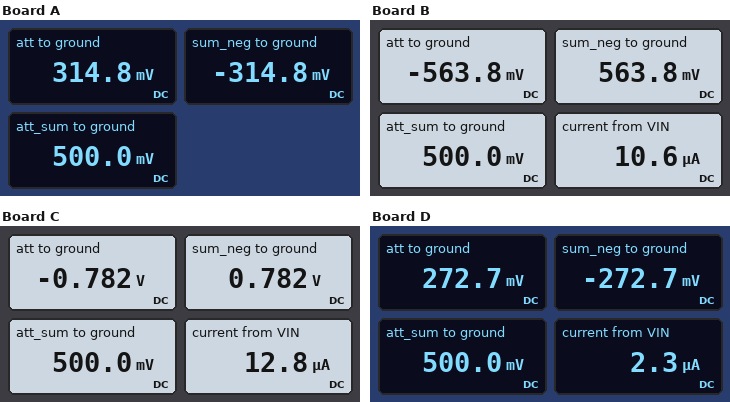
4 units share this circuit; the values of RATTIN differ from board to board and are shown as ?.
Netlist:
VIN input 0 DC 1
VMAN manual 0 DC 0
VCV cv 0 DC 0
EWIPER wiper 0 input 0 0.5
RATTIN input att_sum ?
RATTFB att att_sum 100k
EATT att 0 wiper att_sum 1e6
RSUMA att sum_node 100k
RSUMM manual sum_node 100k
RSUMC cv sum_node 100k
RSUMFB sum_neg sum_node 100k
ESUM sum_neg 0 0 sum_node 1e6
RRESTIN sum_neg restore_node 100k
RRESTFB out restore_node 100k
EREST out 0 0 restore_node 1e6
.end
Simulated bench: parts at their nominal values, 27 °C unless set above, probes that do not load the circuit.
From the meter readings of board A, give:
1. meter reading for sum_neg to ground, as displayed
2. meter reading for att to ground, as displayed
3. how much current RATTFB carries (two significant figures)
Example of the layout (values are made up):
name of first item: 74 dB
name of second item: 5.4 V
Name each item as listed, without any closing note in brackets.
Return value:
meter reading for sum_neg to ground, as displayed: -314.8 mV
meter reading for att to ground, as displayed: 314.8 mV
how much current RATTFB carries: 1.9 µA
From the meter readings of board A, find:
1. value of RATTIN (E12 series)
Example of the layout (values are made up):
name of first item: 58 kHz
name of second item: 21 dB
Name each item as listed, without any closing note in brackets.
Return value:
value of RATTIN: 270 kΩ
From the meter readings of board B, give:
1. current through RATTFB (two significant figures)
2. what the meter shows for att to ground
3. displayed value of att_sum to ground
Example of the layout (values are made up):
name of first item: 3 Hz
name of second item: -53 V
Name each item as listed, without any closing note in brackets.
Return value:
current through RATTFB: 11 µA
what the meter shows for att to ground: -563.8 mV
displayed value of att_sum to ground: 500.0 mV
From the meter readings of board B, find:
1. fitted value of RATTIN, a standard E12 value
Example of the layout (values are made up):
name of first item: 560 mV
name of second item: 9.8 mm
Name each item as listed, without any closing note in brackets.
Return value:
fitted value of RATTIN, a standard E12 value: 47 kΩ
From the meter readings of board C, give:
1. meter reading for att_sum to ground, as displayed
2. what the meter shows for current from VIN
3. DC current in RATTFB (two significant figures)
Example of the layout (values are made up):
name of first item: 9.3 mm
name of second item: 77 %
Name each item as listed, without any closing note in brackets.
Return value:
meter reading for att_sum to ground, as displayed: 500.0 mV
what the meter shows for current from VIN: 12.8 µA
DC current in RATTFB: 13 µA
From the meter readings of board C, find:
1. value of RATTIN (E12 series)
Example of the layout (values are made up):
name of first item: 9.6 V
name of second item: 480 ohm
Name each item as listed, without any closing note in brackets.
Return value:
value of RATTIN: 39 kΩ
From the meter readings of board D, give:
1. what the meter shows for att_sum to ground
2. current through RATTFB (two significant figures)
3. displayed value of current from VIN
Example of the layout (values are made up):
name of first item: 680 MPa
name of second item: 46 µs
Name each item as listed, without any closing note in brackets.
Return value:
what the meter shows for att_sum to ground: 500.0 mV
current through RATTFB: 2.3 µA
displayed value of current from VIN: 2.3 µA
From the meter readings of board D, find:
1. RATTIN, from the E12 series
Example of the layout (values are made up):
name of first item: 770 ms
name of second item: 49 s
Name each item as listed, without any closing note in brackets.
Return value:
RATTIN, from the E12 series: 220 kΩ
